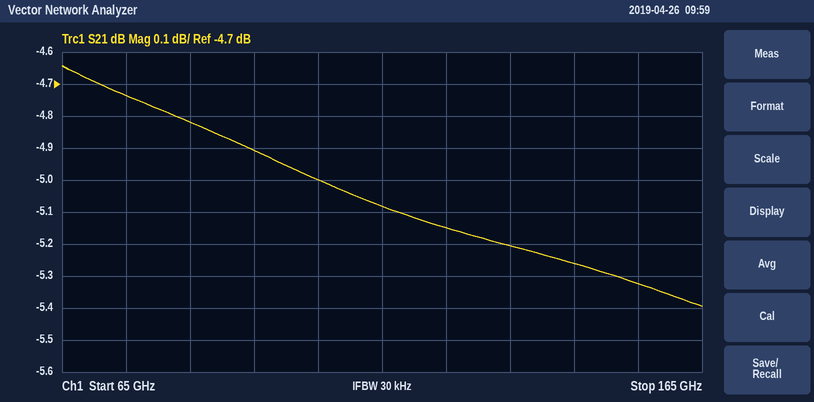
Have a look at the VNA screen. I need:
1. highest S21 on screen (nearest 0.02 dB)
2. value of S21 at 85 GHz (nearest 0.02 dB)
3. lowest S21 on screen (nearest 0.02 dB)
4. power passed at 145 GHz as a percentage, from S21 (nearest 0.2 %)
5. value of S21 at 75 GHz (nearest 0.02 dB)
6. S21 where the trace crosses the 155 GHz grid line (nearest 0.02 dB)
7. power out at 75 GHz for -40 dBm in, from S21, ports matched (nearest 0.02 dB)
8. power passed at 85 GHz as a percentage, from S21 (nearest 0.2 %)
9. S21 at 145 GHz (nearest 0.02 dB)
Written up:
-4.64 dB
-4.82 dB
-5.40 dB
29.8 %
-4.74 dB
-5.32 dB
-44.74 dBm
33.0 %
-5.26 dB
